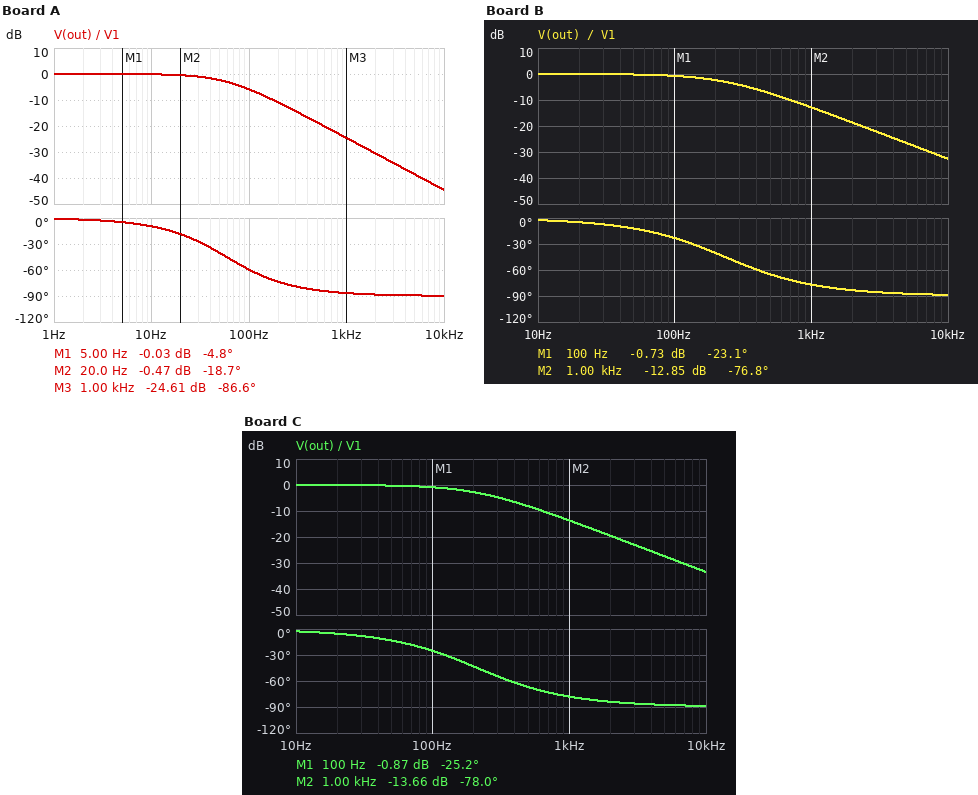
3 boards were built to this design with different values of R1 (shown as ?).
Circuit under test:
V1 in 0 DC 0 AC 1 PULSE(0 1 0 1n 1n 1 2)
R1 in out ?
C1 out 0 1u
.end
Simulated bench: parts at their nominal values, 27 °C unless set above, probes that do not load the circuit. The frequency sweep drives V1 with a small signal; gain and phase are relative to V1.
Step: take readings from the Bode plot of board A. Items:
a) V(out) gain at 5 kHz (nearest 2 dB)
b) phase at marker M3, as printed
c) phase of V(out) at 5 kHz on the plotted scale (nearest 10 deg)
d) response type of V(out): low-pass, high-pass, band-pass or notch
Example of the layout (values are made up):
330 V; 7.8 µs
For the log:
-38 dB; -86.6 deg; -90 deg; low-pass
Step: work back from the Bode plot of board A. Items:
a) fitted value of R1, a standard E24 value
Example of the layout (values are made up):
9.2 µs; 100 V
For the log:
2.7 kΩ
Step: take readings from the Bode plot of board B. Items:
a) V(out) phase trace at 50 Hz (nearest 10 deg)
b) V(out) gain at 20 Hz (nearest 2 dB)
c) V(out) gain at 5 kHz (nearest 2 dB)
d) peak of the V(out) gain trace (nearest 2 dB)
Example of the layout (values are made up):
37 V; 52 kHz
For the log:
-10 deg; 0 dB; -26 dB; 0 dB
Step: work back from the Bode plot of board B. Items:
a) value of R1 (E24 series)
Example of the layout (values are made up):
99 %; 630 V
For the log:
680 Ω
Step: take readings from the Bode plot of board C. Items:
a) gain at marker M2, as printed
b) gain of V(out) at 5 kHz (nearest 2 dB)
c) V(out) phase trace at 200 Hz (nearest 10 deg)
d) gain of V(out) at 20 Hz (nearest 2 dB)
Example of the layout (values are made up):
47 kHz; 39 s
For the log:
-13.66 dB; -28 dB; -40 deg; 0 dB
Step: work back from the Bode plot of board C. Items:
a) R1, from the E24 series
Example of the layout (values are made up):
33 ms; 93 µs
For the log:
750 Ω
